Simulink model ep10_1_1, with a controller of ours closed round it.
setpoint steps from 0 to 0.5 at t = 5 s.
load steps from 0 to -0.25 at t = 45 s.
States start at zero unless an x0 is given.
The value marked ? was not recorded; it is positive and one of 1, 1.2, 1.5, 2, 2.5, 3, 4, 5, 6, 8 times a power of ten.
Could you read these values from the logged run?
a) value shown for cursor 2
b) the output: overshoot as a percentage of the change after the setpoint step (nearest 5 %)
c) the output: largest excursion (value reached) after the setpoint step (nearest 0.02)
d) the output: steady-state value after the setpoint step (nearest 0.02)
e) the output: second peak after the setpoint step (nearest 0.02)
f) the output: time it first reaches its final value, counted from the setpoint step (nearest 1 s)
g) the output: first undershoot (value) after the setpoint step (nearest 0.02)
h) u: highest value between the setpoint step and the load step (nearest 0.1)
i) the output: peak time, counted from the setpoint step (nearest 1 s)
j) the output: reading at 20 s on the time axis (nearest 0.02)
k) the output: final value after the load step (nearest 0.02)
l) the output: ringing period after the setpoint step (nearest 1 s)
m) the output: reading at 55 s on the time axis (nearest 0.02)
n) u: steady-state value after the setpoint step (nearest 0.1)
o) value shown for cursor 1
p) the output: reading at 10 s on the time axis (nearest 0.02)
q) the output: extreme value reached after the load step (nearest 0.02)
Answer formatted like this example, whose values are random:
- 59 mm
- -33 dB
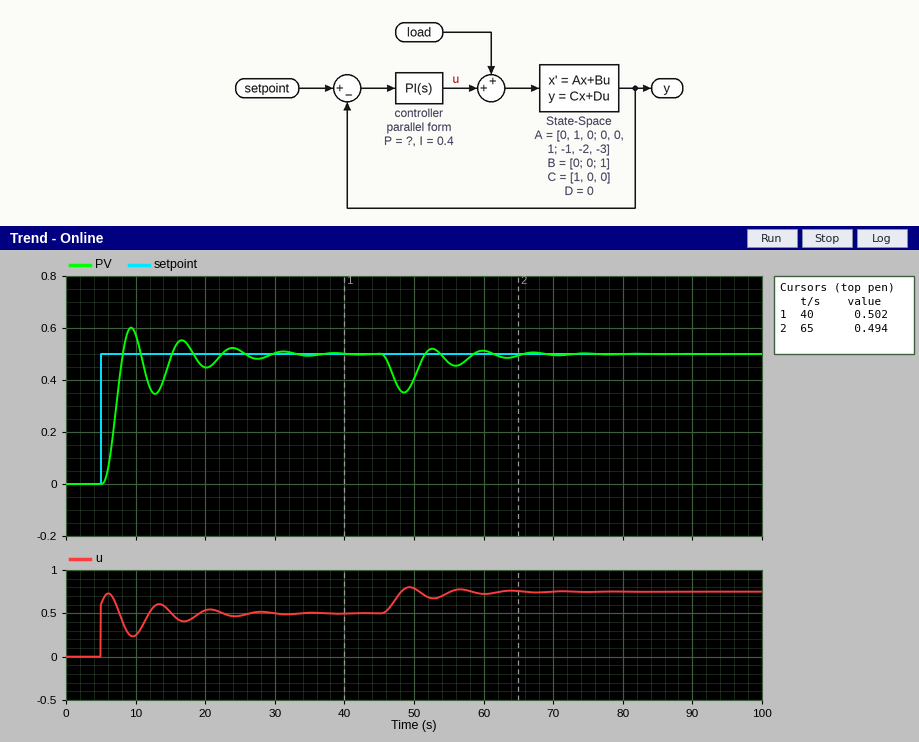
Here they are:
- 0.494
- 20 %
- 0.60
- 0.50
- 0.56
- 3 s
- 0.34
- 0.7
- 4 s
- 0.44
- 0.50
- 7 s
- 0.46
- 0.5
- 0.502
- 0.58
- 0.36
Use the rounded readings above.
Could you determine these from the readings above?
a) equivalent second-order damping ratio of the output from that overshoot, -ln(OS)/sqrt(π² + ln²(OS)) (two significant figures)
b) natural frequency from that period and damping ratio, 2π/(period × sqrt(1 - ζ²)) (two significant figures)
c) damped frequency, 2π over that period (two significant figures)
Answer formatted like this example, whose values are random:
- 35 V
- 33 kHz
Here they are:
- 0.46
- 1.0 rad/s
- 0.90 rad/s
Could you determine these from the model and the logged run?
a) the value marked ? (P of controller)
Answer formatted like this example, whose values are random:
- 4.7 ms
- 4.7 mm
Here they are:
- 1.2
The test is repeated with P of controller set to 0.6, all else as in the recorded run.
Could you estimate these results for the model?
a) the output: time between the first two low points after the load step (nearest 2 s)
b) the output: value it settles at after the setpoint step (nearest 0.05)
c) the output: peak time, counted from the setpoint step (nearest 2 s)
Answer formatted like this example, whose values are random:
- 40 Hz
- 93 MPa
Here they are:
- 10 s
- 0.50
- 6 s
